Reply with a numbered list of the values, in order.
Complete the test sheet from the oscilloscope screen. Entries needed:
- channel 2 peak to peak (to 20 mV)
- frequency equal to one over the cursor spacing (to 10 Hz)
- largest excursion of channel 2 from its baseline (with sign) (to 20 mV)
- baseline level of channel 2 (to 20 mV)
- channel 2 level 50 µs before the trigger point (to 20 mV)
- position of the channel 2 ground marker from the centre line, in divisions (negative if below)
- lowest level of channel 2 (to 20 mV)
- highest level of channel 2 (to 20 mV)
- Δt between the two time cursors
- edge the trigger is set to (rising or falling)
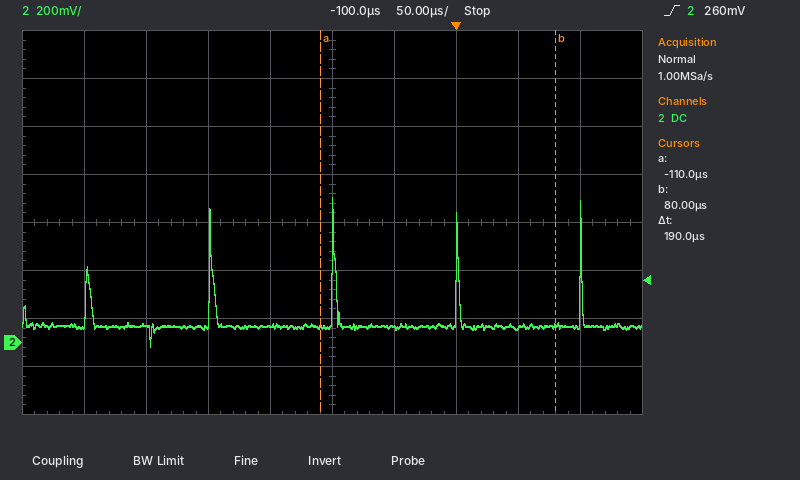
1. 620 mV
2. 5.26 kHz
3. +540 mV
4. 60 mV
5. 60 mV
6. -2.5 div
7. -20 mV
8. 600 mV
9. 190 µs
10. rising
